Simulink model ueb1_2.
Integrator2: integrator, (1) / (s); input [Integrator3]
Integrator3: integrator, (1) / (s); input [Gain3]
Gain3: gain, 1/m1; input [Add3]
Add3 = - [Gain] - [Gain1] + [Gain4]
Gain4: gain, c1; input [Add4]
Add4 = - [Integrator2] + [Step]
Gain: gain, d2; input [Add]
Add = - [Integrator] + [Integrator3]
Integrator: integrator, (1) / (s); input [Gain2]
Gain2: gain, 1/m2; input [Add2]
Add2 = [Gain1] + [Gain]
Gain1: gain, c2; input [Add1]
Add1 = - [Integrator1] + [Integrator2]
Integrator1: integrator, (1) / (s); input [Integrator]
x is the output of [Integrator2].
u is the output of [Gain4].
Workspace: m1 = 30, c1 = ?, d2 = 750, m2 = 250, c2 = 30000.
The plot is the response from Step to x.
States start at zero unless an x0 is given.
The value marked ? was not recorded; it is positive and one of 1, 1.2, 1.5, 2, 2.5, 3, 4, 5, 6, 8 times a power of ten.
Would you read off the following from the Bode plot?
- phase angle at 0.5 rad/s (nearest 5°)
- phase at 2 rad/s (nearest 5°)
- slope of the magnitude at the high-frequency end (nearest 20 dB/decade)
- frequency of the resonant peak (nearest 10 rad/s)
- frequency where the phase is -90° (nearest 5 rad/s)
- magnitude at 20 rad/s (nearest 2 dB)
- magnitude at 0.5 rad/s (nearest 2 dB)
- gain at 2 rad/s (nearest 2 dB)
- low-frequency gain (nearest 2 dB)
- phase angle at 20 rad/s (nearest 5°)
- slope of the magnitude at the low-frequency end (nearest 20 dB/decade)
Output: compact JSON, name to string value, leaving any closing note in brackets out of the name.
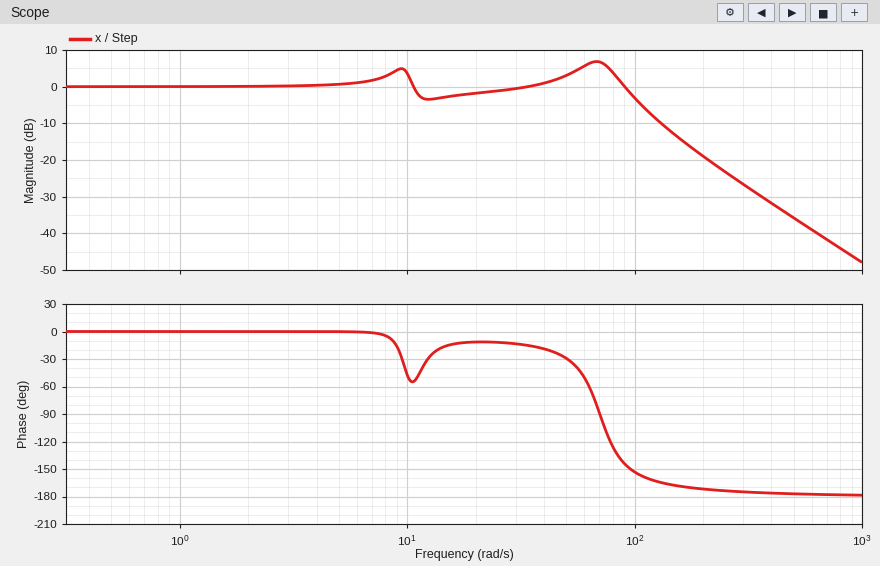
{"phase angle at 0.5 rad/s": "0°", "phase at 2 rad/s": "0°", "slope of the magnitude at the high-frequency end": "-40 dB/decade", "frequency of the resonant peak": "70 rad/s", "frequency where the phase is -90°": "70 rad/s", "magnitude at 20 rad/s": "-2 dB", "magnitude at 0.5 rad/s": "0 dB", "gain at 2 rad/s": "0 dB", "low-frequency gain": "0 dB", "phase angle at 20 rad/s": "-10°", "slope of the magnitude at the low-frequency end": "0 dB/decade"}
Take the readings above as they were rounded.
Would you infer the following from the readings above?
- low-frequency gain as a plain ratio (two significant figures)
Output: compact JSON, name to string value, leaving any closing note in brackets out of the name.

{"low-frequency gain as a plain ratio": "1.0"}
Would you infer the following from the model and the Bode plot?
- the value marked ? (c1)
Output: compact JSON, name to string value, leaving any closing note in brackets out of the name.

{"the value marked ?": "120000"}
